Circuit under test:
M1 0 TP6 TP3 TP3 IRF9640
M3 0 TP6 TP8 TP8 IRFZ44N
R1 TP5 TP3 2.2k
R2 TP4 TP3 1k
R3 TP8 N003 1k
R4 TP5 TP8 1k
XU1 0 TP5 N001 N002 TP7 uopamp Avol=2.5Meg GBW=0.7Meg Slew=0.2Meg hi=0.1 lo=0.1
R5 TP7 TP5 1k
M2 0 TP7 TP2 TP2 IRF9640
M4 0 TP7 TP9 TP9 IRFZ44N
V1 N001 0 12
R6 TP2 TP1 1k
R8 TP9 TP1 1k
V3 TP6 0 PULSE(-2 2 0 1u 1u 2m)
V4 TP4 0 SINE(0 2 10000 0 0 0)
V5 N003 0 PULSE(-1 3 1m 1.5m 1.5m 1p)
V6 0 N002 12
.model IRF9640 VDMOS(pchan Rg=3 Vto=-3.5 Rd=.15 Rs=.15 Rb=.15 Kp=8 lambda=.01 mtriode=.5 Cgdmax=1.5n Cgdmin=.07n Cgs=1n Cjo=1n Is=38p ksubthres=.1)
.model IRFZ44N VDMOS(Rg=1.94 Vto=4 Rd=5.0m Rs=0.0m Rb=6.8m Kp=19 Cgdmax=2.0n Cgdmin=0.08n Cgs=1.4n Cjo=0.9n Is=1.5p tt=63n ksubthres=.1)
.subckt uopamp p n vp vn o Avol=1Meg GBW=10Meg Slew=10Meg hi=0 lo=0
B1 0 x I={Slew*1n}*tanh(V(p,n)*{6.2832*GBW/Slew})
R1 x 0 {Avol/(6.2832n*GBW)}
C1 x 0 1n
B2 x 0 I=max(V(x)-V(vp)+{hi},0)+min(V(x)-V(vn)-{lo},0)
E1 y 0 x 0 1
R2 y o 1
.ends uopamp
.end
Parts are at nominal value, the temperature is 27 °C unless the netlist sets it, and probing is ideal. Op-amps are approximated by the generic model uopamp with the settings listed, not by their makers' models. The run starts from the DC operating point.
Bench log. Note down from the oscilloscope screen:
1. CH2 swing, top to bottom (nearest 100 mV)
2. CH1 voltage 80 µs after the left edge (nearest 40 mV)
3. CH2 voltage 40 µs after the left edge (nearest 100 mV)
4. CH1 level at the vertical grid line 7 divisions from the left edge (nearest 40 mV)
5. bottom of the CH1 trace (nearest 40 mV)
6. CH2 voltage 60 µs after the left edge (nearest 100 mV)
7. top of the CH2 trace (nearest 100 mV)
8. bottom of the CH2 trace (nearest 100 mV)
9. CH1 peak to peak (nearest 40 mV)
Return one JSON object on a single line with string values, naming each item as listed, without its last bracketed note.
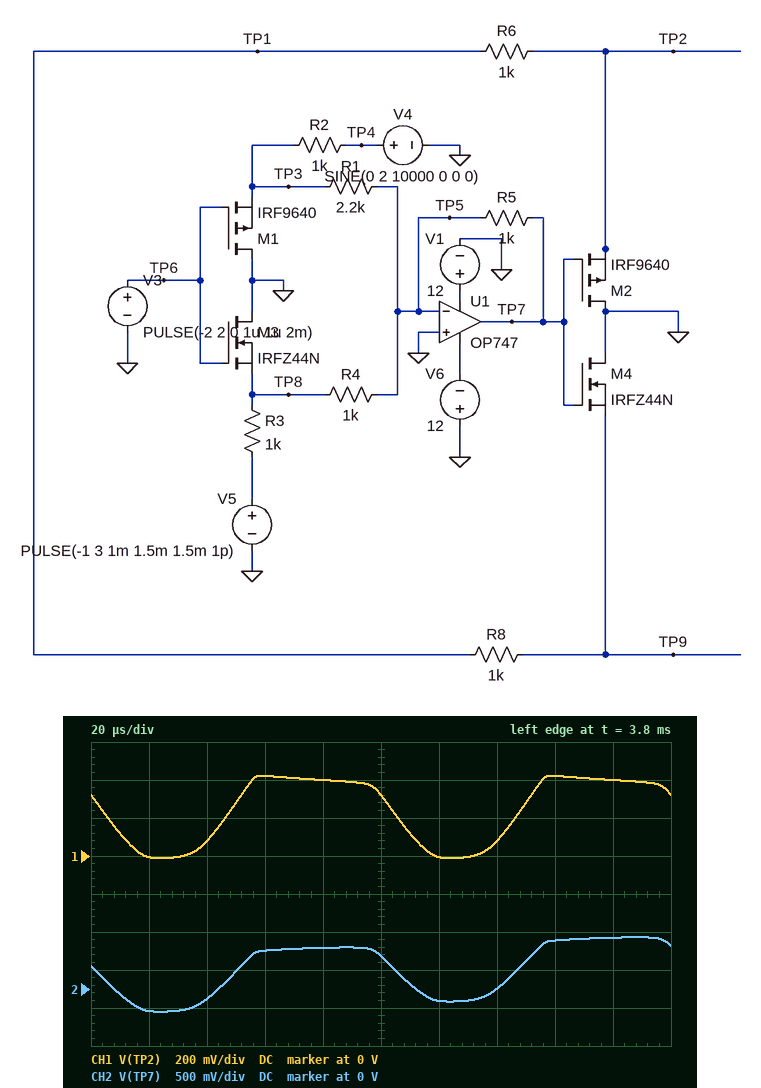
{"CH2 swing, top to bottom": "1.0 V", "CH1 voltage 80 µs after the left edge": "400 mV", "CH2 voltage 40 µs after the left edge": "-100 mV", "CH1 level at the vertical grid line 7 divisions from the left edge": "80 mV", "bottom of the CH1 trace": "0 V", "CH2 voltage 60 µs after the left edge": "500 mV", "top of the CH2 trace": "700 mV", "bottom of the CH2 trace": "-300 mV", "CH1 peak to peak": "440 mV"}
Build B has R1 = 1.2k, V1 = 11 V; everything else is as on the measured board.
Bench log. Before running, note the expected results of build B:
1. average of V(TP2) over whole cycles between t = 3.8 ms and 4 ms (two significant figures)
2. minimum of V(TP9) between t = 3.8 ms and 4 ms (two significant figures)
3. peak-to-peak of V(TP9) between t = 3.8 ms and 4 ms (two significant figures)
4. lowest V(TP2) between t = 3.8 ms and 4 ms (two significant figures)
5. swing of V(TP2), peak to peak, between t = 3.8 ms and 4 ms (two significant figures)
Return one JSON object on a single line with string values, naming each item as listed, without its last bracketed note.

{"average of V(TP2) over whole cycles between t = 3.8 ms and 4 ms": "140 mV", "minimum of V(TP9) between t = 3.8 ms and 4 ms": "-290 mV", "peak-to-peak of V(TP9) between t = 3.8 ms and 4 ms": "700 mV", "lowest V(TP2) between t = 3.8 ms and 4 ms": "-280 mV", "swing of V(TP2), peak to peak, between t = 3.8 ms and 4 ms": "710 mV"}
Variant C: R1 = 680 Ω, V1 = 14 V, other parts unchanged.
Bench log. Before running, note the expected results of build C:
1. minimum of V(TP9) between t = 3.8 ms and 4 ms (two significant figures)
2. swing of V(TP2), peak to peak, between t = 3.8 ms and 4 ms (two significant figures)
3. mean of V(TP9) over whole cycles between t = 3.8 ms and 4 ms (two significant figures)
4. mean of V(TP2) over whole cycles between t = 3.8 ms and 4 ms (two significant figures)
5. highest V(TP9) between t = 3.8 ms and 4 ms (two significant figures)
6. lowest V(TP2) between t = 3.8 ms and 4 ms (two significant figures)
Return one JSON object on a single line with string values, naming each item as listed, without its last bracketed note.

{"minimum of V(TP9) between t = 3.8 ms and 4 ms": "-460 mV", "swing of V(TP2), peak to peak, between t = 3.8 ms and 4 ms": "930 mV", "mean of V(TP9) over whole cycles between t = 3.8 ms and 4 ms": "86 mV", "mean of V(TP2) over whole cycles between t = 3.8 ms and 4 ms": "110 mV", "highest V(TP9) between t = 3.8 ms and 4 ms": "470 mV", "lowest V(TP2) between t = 3.8 ms and 4 ms": "-380 mV"}
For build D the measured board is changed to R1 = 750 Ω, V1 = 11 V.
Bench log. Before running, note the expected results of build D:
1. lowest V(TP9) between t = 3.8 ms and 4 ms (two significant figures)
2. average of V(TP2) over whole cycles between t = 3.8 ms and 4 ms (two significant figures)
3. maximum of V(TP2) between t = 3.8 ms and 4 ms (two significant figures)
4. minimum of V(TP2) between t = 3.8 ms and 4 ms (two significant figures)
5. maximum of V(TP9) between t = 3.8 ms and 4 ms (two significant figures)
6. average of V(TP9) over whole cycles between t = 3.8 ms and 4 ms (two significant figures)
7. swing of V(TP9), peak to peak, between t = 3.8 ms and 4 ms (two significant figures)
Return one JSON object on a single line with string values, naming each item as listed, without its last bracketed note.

{"lowest V(TP9) between t = 3.8 ms and 4 ms": "-440 mV", "average of V(TP2) over whole cycles between t = 3.8 ms and 4 ms": "110 mV", "maximum of V(TP2) between t = 3.8 ms and 4 ms": "530 mV", "minimum of V(TP2) between t = 3.8 ms and 4 ms": "-370 mV", "maximum of V(TP9) between t = 3.8 ms and 4 ms": "470 mV", "average of V(TP9) over whole cycles between t = 3.8 ms and 4 ms": "93 mV", "swing of V(TP9), peak to peak, between t = 3.8 ms and 4 ms": "910 mV"}
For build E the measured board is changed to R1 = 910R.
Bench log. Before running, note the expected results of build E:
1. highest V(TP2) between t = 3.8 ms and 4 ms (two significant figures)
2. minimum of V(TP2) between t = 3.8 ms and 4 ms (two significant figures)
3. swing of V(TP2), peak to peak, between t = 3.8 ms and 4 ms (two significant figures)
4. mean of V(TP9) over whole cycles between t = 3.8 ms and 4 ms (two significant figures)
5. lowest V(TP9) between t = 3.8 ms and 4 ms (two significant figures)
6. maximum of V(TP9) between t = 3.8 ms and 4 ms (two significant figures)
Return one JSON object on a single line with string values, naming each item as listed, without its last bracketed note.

{"highest V(TP2) between t = 3.8 ms and 4 ms": "480 mV", "minimum of V(TP2) between t = 3.8 ms and 4 ms": "-350 mV", "swing of V(TP2), peak to peak, between t = 3.8 ms and 4 ms": "840 mV", "mean of V(TP9) over whole cycles between t = 3.8 ms and 4 ms": "110 mV", "lowest V(TP9) between t = 3.8 ms and 4 ms": "-390 mV", "maximum of V(TP9) between t = 3.8 ms and 4 ms": "450 mV"}
